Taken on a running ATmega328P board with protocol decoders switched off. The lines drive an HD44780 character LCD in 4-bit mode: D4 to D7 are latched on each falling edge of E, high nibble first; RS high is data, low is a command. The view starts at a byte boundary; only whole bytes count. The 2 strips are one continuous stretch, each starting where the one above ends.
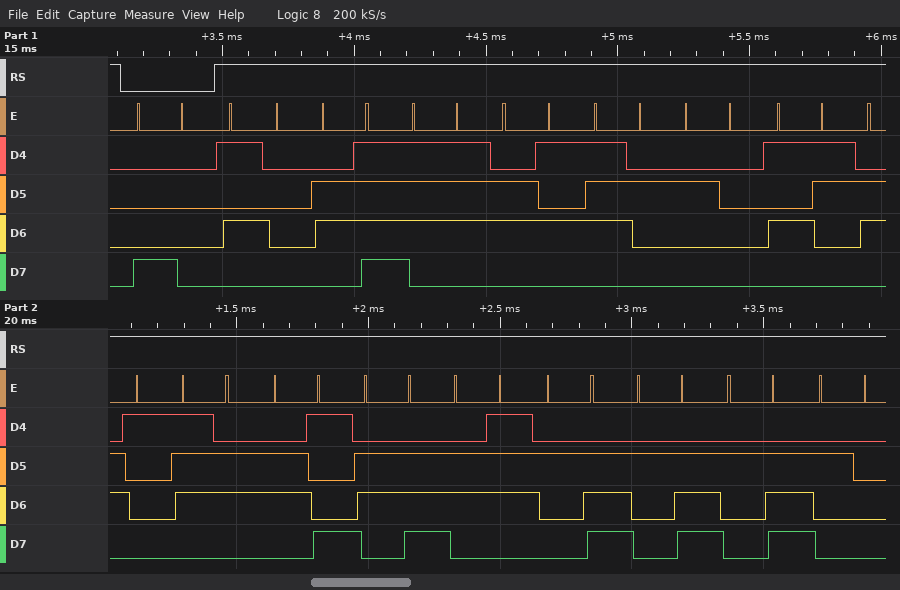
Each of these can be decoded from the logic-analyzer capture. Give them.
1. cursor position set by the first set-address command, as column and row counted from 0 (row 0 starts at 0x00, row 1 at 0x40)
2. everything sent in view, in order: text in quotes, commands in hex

column 0, row 0
0x80 "Power Saving... "
